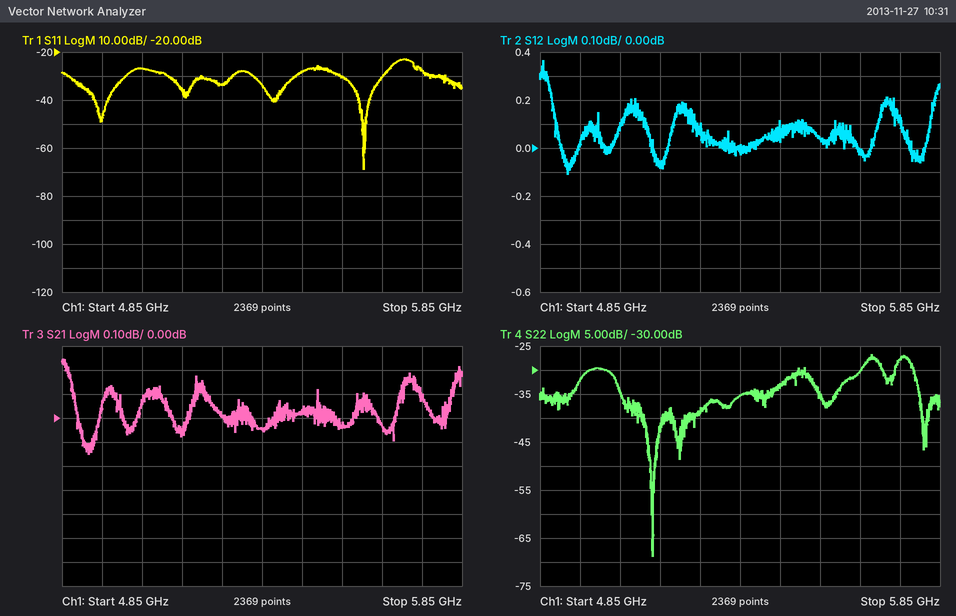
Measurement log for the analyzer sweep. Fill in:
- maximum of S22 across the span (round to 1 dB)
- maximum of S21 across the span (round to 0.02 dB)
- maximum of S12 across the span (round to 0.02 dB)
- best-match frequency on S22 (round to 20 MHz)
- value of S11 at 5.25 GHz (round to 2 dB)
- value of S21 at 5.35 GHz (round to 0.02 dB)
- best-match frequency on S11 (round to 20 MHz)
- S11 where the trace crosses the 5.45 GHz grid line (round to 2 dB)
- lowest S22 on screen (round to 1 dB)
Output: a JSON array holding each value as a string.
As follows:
["-27 dB", "0.24 dB", "0.36 dB", "5.14 GHz", "-34 dB", "-0.04 dB", "5.60 GHz", "-28 dB", "-69 dB"]
